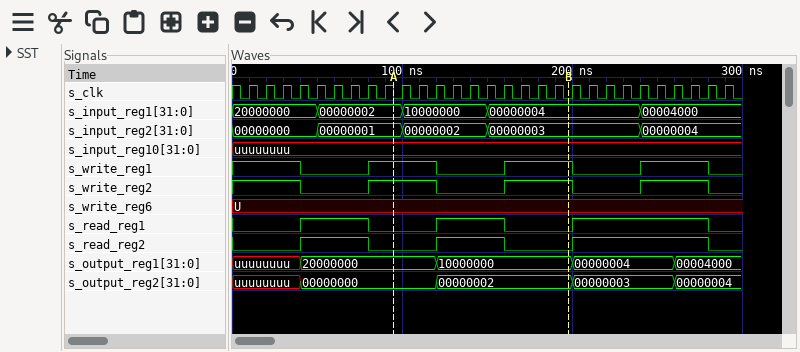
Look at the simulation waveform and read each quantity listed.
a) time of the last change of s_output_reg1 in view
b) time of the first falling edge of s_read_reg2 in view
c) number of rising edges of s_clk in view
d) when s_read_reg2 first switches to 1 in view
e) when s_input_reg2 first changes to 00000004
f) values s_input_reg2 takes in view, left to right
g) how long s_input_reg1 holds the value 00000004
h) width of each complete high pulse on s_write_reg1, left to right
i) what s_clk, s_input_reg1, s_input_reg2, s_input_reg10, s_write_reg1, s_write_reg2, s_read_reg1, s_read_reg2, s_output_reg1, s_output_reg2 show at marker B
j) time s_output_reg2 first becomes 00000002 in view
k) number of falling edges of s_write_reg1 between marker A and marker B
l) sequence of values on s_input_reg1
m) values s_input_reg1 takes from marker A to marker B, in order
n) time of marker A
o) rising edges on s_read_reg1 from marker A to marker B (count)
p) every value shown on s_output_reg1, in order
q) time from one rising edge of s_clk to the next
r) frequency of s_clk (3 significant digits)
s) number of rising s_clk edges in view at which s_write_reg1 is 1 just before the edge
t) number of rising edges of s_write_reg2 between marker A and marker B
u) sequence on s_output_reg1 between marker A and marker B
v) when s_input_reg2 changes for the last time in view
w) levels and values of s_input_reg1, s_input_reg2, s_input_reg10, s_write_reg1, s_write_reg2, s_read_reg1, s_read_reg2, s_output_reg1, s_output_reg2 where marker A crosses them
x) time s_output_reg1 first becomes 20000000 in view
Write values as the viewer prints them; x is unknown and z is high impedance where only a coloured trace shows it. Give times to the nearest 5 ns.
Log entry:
260 ns
80 ns
29
40 ns
240 ns
00000000, 00000001, 00000002, 00000003, 00000004
90 ns
40 ns, 40 ns, 40 ns
s_clk=0, s_input_reg1=00000004, s_input_reg2=00000003, s_input_reg10=uuuuuuuu, s_write_reg1=1, s_write_reg2=1, s_read_reg1=0, s_read_reg2=0, s_output_reg1=10000000, s_output_reg2=00000002
120 ns
1
20000000, 00000002, 10000000, 00000004, 00004000
00000002, 10000000, 00000004
95 ns
1
uuuuuuuu, 20000000, 10000000, 00000004, 00004000
10 ns
100 MHz
16
1
20000000, 10000000
240 ns
s_input_reg1=00000002, s_input_reg2=00000001, s_input_reg10=uuuuuuuu, s_write_reg1=1, s_write_reg2=1, s_read_reg1=0, s_read_reg2=0, s_output_reg1=20000000, s_output_reg2=00000000
40 ns
